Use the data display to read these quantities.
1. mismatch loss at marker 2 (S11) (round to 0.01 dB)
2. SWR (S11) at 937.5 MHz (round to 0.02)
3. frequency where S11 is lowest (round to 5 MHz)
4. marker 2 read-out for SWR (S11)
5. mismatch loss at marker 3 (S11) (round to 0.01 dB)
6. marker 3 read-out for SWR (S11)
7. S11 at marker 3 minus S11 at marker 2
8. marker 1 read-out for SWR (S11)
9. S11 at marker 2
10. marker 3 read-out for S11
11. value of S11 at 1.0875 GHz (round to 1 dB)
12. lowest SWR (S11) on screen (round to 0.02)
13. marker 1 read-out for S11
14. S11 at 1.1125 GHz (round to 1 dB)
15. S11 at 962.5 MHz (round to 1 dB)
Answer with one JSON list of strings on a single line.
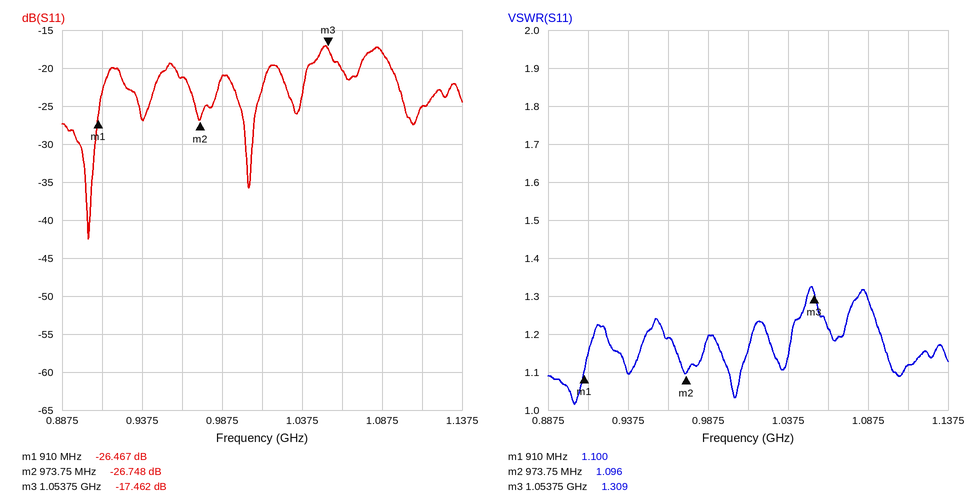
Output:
["0.01 dB", "1.10", "905 MHz", "1.096", "0.08 dB", "1.309", "9.286 dB", "1.100", "-26.748 dB", "-17.462 dB", "-18 dB", "1.02", "-26.467 dB", "-25 dB", "-21 dB"]
